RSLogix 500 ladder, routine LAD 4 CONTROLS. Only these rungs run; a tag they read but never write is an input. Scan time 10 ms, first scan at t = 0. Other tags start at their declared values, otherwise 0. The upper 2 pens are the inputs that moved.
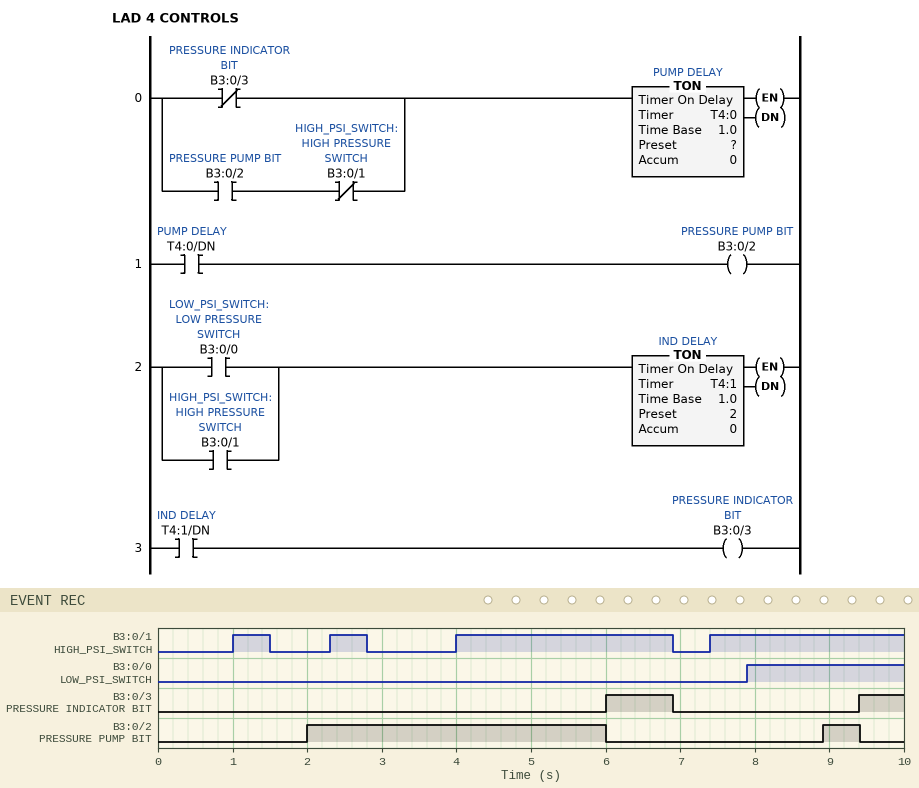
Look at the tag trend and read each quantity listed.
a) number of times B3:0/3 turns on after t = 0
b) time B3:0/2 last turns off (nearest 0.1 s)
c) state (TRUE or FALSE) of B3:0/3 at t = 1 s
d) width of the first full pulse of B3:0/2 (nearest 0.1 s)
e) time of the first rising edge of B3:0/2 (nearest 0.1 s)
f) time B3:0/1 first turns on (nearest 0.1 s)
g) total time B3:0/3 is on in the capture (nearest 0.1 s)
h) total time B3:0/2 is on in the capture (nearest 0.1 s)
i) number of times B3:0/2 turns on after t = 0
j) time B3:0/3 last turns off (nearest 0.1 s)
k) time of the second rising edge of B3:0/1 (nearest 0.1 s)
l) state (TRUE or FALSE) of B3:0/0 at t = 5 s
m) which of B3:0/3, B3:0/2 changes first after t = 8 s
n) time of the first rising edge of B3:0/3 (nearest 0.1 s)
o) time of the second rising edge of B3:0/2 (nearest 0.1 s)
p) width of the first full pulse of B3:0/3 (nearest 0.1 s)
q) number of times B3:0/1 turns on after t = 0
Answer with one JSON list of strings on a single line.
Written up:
["2", "9.4 s", "FALSE", "4.0 s", "2.0 s", "1.0 s", "1.5 s", "4.5 s", "2", "6.9 s", "2.3 s", "FALSE", "B3:0/2", "6.0 s", "8.9 s", "0.9 s", "4"]
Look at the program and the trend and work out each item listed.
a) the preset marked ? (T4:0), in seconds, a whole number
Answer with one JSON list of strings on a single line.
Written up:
["2 s"]
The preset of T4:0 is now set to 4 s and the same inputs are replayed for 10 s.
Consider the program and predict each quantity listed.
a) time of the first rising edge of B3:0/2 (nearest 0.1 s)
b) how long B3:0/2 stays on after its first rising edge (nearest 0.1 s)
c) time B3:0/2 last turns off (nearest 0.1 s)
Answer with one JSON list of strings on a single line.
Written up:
["4.0 s", "2.0 s", "6.0 s"]
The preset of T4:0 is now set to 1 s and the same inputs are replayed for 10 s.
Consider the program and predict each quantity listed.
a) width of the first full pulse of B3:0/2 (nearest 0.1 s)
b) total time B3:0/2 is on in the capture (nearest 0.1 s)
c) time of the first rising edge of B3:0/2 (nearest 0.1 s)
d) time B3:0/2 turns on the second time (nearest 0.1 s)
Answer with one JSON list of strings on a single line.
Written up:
["5.0 s", "6.5 s", "1.0 s", "7.9 s"]
